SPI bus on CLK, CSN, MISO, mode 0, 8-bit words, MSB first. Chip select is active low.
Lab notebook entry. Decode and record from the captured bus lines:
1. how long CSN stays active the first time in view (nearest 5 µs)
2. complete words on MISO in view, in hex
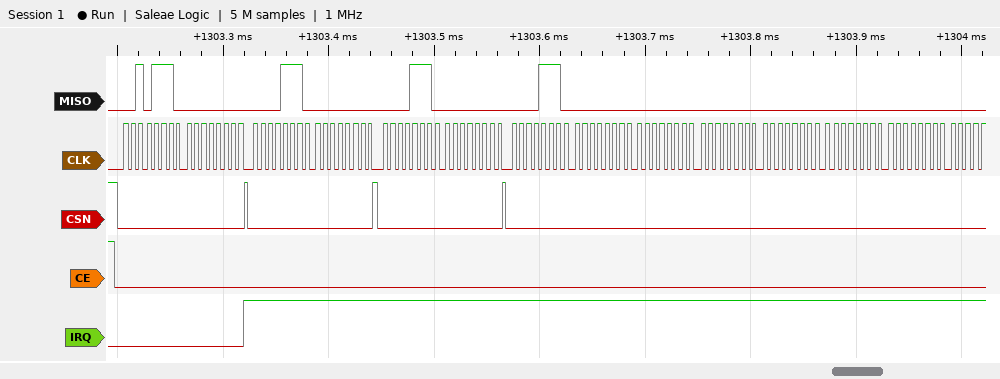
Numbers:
120 µs
2E, 00, 0E, 00, 0E, 00, 0E, 00, 00, 00, 00, 00, 00
